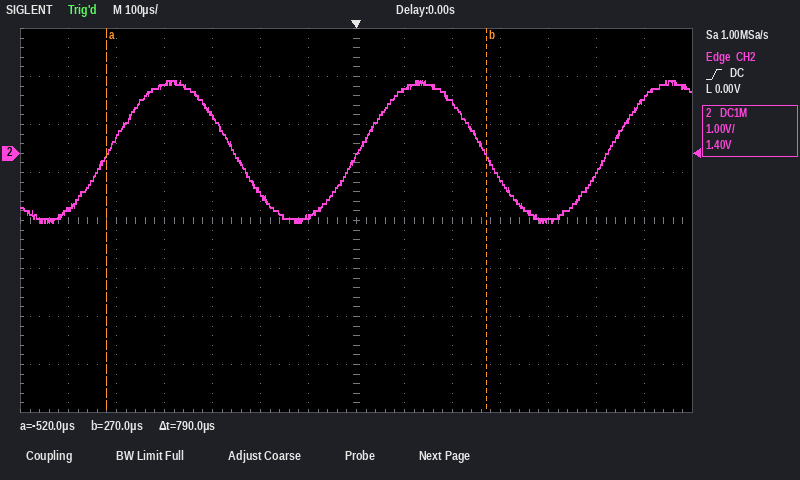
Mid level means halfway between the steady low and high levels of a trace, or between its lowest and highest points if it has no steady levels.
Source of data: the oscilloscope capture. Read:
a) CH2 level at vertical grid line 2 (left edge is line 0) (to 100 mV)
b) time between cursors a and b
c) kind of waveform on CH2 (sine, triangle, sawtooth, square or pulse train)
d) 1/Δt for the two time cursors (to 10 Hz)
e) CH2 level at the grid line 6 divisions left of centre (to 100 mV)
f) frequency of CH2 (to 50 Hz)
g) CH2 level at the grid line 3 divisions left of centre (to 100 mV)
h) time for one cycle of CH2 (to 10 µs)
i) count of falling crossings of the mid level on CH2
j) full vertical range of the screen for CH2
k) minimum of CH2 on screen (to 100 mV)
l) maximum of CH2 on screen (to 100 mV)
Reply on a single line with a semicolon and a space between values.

300 mV; 790 µs; sine; 1.27 kHz; -1.2 V; 1.90 kHz; 800 mV; 520 µs; 2; 8 V; -1.4 V; 1.5 V
